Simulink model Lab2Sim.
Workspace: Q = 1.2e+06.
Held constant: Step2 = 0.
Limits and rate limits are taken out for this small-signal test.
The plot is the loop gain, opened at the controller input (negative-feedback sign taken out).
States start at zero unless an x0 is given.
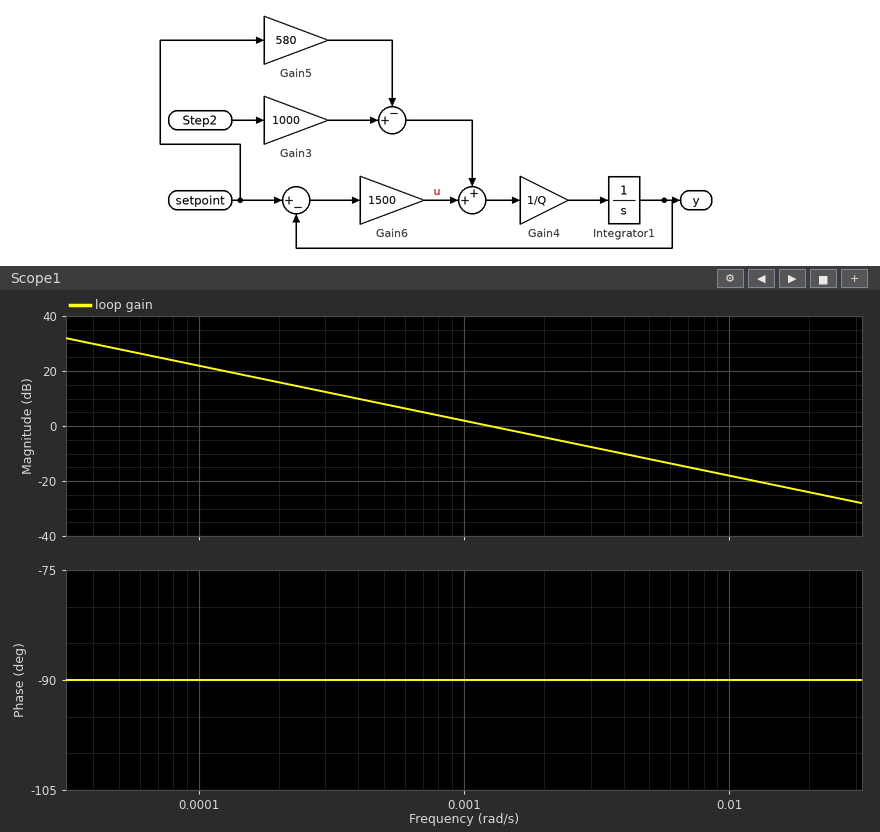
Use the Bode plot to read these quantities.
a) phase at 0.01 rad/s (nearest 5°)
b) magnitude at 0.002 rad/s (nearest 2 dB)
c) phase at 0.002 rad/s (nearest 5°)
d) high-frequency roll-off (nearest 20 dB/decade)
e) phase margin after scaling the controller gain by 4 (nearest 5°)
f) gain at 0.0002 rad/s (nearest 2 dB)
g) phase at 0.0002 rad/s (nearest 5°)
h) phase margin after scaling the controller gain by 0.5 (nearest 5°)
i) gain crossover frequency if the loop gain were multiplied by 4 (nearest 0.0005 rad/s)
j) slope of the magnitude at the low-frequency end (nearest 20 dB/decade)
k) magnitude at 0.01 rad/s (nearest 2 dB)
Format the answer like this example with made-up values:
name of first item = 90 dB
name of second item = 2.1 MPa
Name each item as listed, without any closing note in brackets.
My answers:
phase at 0.01 rad/s = -90°
magnitude at 0.002 rad/s = -4 dB
phase at 0.002 rad/s = -90°
high-frequency roll-off = -20 dB/decade
phase margin after scaling the controller gain by 4 = 90°
gain at 0.0002 rad/s = 16 dB
phase at 0.0002 rad/s = -90°
phase margin after scaling the controller gain by 0.5 = 90°
gain crossover frequency if the loop gain were multiplied by 4 = 0.0050 rad/s
slope of the magnitude at the low-frequency end = -20 dB/decade
magnitude at 0.01 rad/s = -18 dB
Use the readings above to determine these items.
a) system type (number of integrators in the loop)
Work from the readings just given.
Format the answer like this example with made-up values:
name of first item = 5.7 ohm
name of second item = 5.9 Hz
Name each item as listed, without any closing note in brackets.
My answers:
system type = 1
